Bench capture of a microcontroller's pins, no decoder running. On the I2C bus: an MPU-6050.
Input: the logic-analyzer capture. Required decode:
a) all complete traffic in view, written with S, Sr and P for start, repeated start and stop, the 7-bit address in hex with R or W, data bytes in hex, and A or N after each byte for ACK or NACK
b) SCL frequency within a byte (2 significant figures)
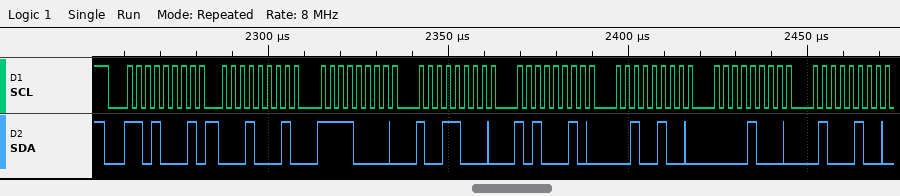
S 68R A 11 A F0 A 98 A A2 A 24 A 08 A 44 A
400 kHz
